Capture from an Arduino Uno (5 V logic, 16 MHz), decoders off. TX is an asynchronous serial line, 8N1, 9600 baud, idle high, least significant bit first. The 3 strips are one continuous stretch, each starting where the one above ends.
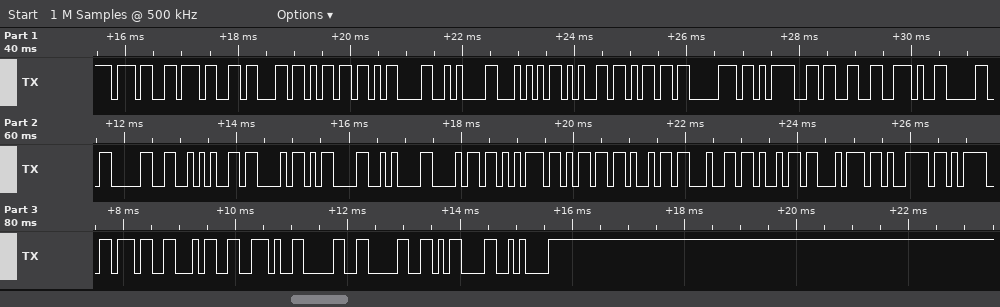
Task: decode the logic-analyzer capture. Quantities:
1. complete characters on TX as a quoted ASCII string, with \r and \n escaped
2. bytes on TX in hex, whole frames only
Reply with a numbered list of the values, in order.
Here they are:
1. "77cm\r\nTemp=3.00*C\r\nhumidity=74.00\r\n"
2. 0x37 0x37 0x63 0x6D 0x0D 0x0A 0x54 0x65 0x6D 0x70 0x3D 0x33 0x2E 0x30 0x30 0x2A 0x43 0x0D 0x0A 0x68 0x75 0x6D 0x69 0x64 0x69 0x74 0x79 0x3D 0x37 0x34 0x2E 0x30 0x30 0x0D 0x0A
